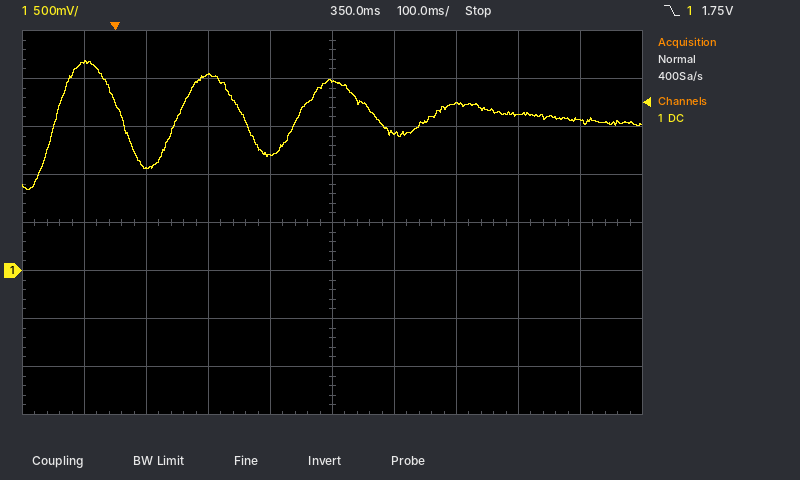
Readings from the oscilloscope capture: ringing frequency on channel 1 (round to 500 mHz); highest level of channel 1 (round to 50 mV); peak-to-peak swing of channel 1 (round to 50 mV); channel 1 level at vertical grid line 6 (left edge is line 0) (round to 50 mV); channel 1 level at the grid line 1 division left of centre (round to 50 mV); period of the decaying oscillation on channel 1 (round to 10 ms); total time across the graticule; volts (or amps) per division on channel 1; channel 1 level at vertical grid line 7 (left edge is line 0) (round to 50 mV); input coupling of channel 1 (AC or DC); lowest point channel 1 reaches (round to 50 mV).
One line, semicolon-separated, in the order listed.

5.0 Hz; 2.20 V; 1.35 V; 1.45 V; 1.20 V; 200 ms; 1 s; 500 mV; 1.75 V; DC; 850 mV
